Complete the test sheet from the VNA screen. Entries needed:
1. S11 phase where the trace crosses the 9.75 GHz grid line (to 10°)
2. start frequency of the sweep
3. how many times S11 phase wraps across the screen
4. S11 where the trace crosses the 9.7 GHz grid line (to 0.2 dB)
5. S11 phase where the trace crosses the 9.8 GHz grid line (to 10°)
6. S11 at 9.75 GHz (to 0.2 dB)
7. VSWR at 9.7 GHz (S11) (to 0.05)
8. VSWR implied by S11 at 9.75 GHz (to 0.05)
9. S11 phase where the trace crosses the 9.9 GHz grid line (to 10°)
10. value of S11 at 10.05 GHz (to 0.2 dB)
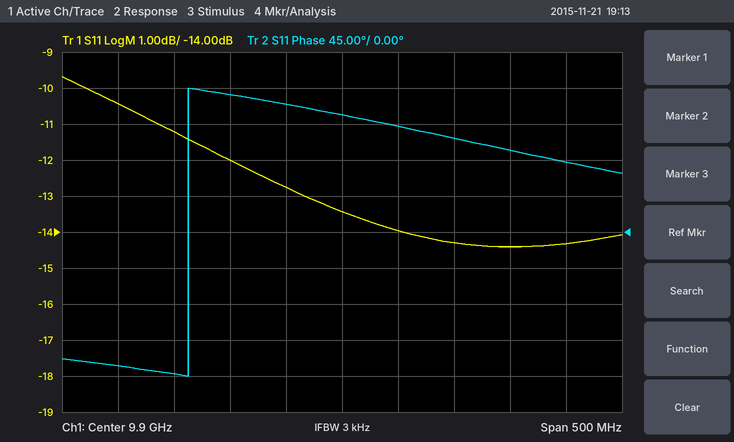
-180°
9.65 GHz
1
-10.4 dB
170°
-11.2 dB
1.85
1.75
150°
-14.4 dB
